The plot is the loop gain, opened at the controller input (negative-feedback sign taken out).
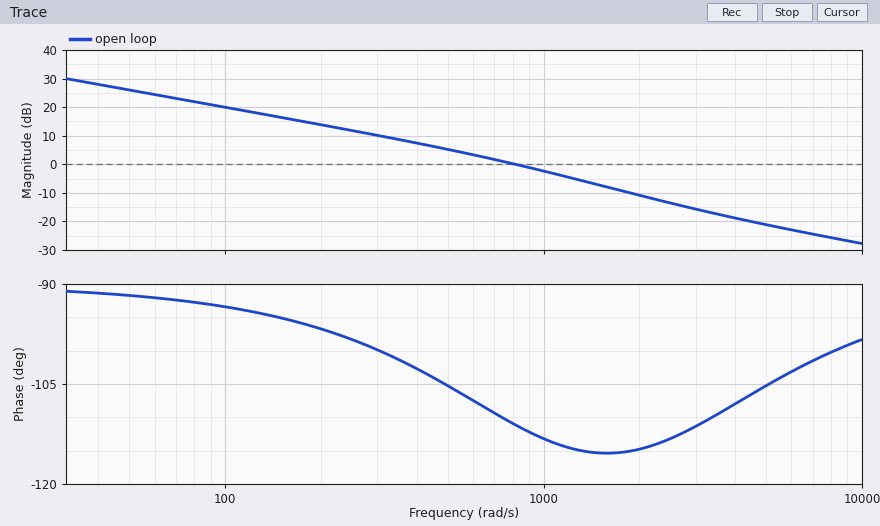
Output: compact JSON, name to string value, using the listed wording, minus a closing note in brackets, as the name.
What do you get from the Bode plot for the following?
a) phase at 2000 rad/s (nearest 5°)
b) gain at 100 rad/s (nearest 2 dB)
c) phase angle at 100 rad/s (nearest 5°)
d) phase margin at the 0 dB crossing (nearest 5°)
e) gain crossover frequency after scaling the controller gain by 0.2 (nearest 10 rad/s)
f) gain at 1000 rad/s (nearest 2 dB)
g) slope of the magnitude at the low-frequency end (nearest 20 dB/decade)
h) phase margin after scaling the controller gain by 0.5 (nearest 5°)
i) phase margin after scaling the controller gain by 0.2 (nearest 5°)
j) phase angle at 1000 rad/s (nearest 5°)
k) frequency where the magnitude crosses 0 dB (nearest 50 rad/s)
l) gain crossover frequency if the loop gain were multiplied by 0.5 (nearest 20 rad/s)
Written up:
{"phase at 2000 rad/s": "-115°", "gain at 100 rad/s": "20 dB", "phase angle at 100 rad/s": "-95°", "phase margin at the 0 dB crossing": "70°", "gain crossover frequency after scaling the controller gain by 0.2": "200 rad/s", "gain at 1000 rad/s": "-2 dB", "slope of the magnitude at the low-frequency end": "-20 dB/decade", "phase margin after scaling the controller gain by 0.5": "75°", "phase margin after scaling the controller gain by 0.2": "85°", "phase angle at 1000 rad/s": "-115°", "frequency where the magnitude crosses 0 dB": "800 rad/s", "gain crossover frequency if the loop gain were multiplied by 0.5": "460 rad/s"}
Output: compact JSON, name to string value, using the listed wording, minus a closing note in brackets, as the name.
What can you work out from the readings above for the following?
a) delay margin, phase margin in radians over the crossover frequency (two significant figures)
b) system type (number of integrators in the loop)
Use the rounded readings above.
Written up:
{"delay margin, phase margin in radians over the crossover frequency": "0.0015 s", "system type": "1"}
